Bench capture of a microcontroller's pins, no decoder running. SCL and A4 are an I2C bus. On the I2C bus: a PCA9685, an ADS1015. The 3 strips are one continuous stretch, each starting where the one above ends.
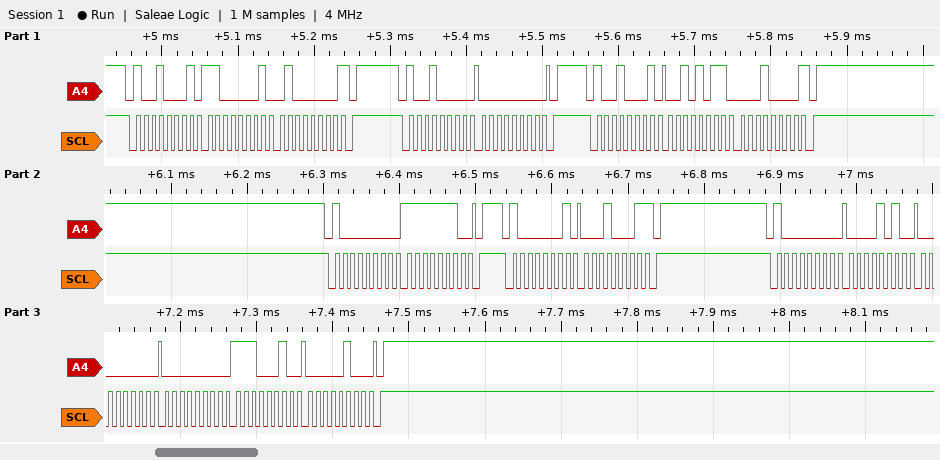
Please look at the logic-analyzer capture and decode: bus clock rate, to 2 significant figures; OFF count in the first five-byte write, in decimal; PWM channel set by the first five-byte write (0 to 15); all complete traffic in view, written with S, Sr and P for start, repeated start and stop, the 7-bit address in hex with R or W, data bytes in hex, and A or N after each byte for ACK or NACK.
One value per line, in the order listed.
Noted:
100 kHz
1250
1
S 48R A C1 A 40 N P S 48W A 00 A P S 48R A 2B A 10 N P S 40W A FE A P S 40R A 11 N P S 40W A 0A A 00 A 00 A E2 A 04 A P
